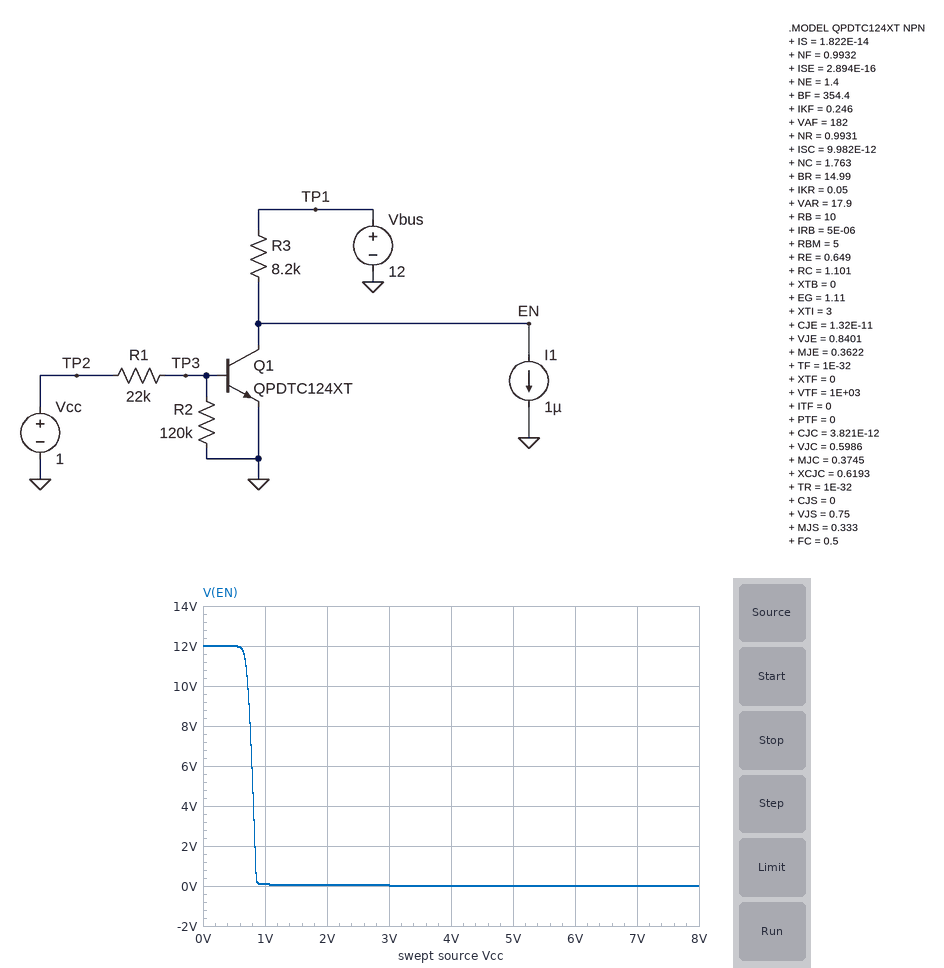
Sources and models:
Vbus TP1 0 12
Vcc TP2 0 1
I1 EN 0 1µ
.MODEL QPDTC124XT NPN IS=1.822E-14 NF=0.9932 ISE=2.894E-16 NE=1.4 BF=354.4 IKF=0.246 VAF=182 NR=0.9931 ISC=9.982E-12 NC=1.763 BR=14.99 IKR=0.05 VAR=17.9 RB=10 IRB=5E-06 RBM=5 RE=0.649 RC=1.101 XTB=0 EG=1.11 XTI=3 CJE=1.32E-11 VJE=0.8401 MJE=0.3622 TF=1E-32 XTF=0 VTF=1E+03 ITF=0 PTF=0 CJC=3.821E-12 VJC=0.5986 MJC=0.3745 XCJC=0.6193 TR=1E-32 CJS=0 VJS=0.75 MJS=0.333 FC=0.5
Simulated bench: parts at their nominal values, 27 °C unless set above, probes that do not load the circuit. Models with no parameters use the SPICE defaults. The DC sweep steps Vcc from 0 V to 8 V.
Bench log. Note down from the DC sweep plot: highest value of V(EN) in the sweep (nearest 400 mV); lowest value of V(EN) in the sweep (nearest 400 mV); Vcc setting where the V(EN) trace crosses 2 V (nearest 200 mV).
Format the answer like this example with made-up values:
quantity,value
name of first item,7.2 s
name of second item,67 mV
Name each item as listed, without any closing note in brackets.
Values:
quantity,value
highest value of V(EN) in the sweep,12.0 V
lowest value of V(EN) in the sweep,0 V
Vcc setting where the V(EN) trace crosses 2 V,800 mV
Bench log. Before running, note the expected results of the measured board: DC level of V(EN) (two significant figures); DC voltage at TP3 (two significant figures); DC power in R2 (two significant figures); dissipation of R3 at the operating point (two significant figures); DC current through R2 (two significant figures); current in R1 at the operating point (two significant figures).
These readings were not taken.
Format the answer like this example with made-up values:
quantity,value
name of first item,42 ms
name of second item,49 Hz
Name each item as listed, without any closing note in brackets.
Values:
quantity,value
DC level of V(EN),88 mV
DC voltage at TP3,650 mV
DC power in R2,3.5 µW
dissipation of R3 at the operating point,17 mW
DC current through R2,5.4 µA
current in R1 at the operating point,16 µA
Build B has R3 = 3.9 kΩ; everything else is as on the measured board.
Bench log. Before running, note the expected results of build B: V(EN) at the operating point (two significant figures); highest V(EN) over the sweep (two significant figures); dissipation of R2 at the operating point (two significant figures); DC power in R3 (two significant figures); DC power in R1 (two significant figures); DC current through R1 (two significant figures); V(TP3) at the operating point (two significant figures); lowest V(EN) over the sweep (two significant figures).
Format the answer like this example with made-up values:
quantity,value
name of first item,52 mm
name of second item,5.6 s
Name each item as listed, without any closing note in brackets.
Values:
quantity,value
V(EN) at the operating point,190 mV
highest V(EN) over the sweep,12 V
dissipation of R2 at the operating point,3.7 µW
DC power in R3,36 mW
DC power in R1,5.0 µW
DC current through R1,15 µA
V(TP3) at the operating point,670 mV
lowest V(EN) over the sweep,23 mV
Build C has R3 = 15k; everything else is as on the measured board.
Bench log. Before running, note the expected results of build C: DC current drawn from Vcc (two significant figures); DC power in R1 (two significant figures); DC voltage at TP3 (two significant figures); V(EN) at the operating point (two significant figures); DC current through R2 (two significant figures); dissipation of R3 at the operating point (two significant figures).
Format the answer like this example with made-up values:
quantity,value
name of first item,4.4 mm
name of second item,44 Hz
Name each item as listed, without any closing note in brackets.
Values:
quantity,value
DC current drawn from Vcc,17 µA
DC power in R1,6.1 µW
DC voltage at TP3,630 mV
V(EN) at the operating point,62 mV
DC current through R2,5.3 µA
dissipation of R3 at the operating point,9.5 mW
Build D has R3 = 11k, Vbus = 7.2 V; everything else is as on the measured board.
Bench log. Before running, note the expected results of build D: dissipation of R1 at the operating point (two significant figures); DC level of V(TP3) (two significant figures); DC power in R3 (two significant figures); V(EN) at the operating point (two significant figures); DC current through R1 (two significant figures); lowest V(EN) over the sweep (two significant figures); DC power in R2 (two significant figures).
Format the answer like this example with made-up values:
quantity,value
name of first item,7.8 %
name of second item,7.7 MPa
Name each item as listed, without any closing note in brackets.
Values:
quantity,value
dissipation of R1 at the operating point,6.2 µW
DC level of V(TP3),630 mV
DC power in R3,4.6 mW
V(EN) at the operating point,55 mV
DC current through R1,17 µA
lowest V(EN) over the sweep,7.3 mV
DC power in R2,3.3 µW
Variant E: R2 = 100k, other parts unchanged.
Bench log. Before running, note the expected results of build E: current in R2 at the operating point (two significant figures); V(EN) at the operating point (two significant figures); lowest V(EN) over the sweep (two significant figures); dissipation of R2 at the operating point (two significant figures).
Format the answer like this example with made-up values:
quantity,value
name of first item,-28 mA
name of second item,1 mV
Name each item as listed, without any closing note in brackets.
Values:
quantity,value
current in R2 at the operating point,6.5 µA
V(EN) at the operating point,93 mV
lowest V(EN) over the sweep,13 mV
dissipation of R2 at the operating point,4.2 µW
